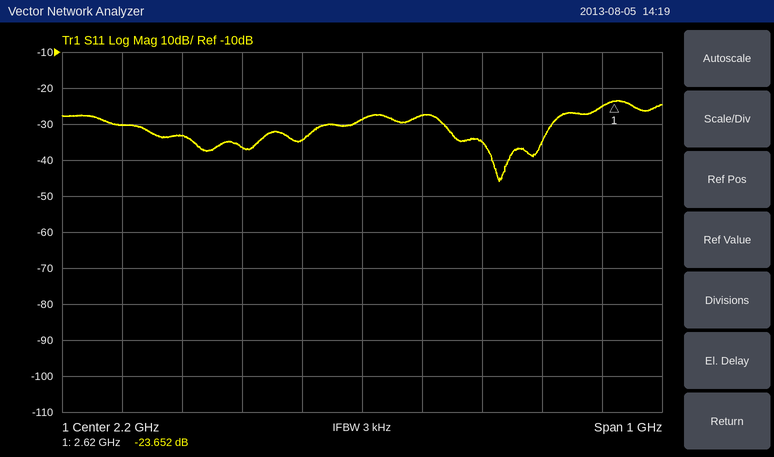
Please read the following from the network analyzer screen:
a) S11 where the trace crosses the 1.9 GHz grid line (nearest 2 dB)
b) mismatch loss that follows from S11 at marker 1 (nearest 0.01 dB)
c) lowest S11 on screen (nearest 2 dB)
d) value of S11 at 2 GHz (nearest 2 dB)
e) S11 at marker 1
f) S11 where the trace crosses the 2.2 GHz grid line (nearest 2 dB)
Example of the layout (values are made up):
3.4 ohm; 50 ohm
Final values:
-34 dB; 0.02 dB; -46 dB; -36 dB; -23.652 dB; -28 dB
